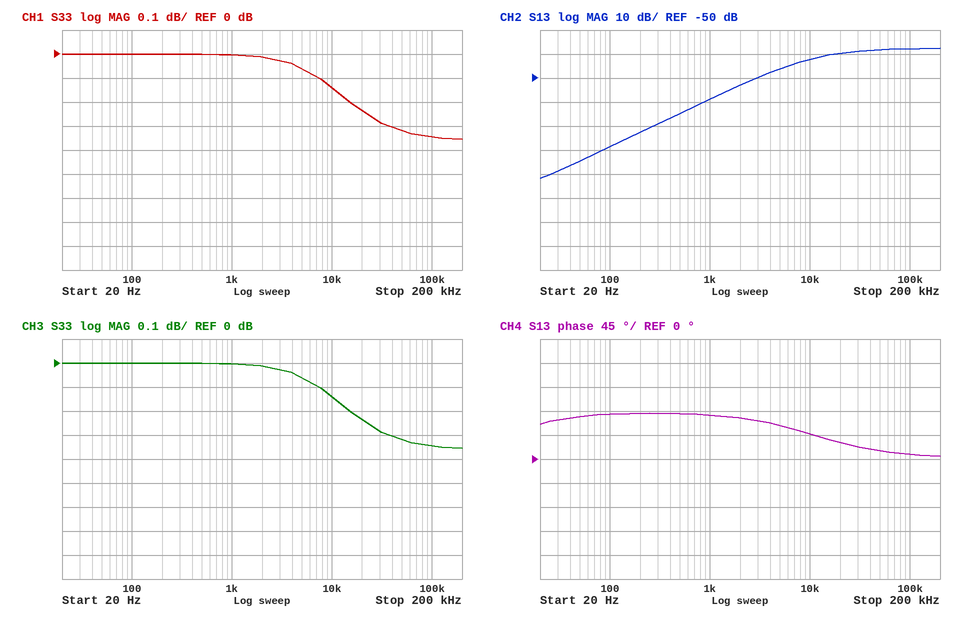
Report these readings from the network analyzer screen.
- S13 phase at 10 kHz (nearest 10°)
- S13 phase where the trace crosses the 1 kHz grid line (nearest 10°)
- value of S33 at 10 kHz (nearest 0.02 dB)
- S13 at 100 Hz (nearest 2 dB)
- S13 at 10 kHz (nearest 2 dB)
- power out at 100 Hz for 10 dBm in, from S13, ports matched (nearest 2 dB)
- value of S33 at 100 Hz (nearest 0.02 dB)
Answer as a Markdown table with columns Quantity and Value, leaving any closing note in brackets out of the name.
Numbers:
| Quantity | Value |
|---|---|
| S13 phase at 10 kHz | 50° |
| S13 phase where the trace crosses the 1 kHz grid line | 80° |
| value of S33 at 10 kHz | -0.14 dB |
| S13 at 100 Hz | -78 dB |
| S13 at 10 kHz | -42 dB |
| power out at 100 Hz for 10 dBm in, from S13, ports matched | -68 dBm |
| value of S33 at 100 Hz | 0.00 dB |
